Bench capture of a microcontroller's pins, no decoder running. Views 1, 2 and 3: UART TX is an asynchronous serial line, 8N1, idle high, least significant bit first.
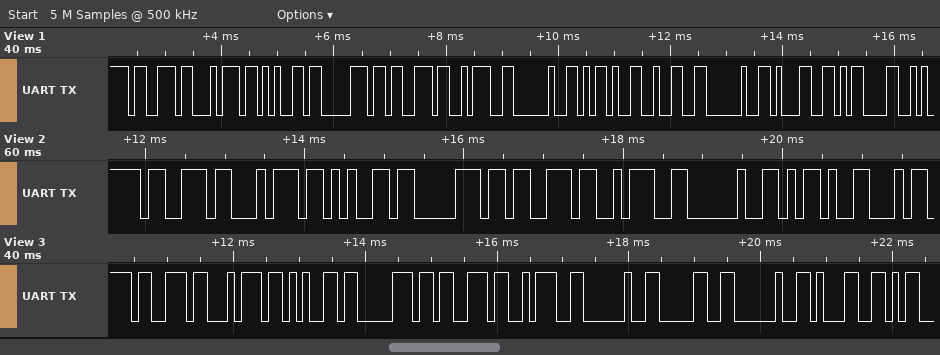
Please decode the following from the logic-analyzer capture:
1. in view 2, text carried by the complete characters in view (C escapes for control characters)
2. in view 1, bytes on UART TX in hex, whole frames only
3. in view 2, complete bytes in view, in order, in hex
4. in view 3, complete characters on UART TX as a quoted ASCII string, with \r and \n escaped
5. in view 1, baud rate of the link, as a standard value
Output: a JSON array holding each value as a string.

["\"steps: -\"", "0x73 0x74 0x65 0x70 0x73 0x3A 0x20 0x2D 0x32 0x20 0x31 0x0D", "73 74 65 70 73 3A 20 2D", "\"steps: 0 1\"", "9600 baud"]
